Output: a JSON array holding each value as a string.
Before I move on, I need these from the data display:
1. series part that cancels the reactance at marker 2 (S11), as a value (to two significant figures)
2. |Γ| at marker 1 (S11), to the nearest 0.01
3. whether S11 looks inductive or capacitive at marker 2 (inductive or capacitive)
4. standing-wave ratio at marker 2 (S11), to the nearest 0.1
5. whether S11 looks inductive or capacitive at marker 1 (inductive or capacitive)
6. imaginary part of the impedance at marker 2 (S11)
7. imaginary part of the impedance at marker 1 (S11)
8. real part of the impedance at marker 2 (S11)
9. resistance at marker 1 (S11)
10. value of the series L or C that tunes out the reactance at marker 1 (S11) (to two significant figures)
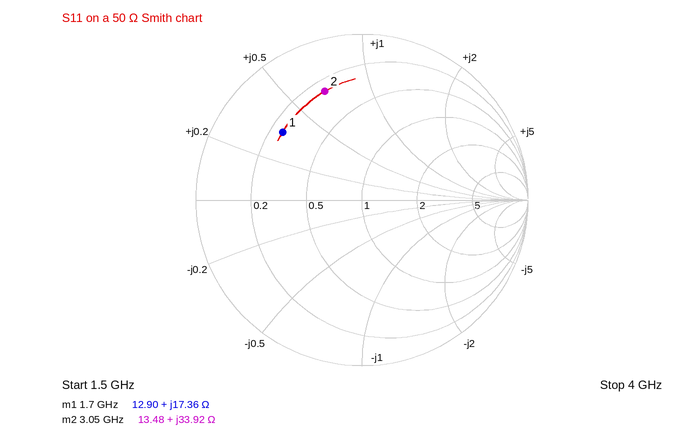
["1.5 pF", "0.63", "inductive", "5.5", "inductive", "+33.92 Ω", "+17.36 Ω", "13.48 Ω", "12.90 Ω", "5.4 pF"]
